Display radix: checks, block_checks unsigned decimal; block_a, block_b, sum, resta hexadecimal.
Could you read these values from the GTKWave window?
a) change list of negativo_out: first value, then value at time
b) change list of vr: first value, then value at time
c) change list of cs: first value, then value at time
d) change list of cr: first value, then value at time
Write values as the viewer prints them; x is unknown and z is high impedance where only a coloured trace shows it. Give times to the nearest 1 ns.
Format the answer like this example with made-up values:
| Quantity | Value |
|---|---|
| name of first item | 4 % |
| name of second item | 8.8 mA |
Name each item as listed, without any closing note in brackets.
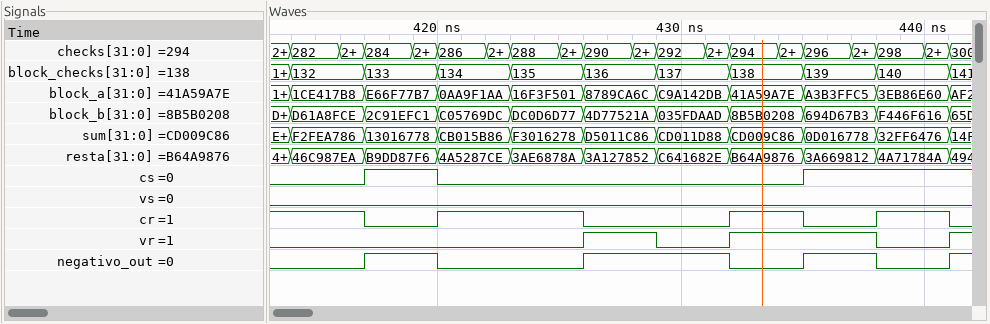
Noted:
| Quantity | Value |
|---|---|
| change list of negativo_out: first value, then value at time | 0, 1 at 417 ns, 0 at 420 ns, 1 at 426 ns, 0 at 432 ns, 1 at 435 ns, 0 at 438 ns, 1 at 441 ns |
| change list of vr: first value, then value at time | 0, 1 at 426 ns, 0 at 429 ns, 1 at 432 ns, 0 at 438 ns, 1 at 441 ns |
| change list of cs: first value, then value at time | 0, 1 at 417 ns, 0 at 420 ns, 1 at 435 ns |
| change list of cr: first value, then value at time | 1, 0 at 417 ns, 1 at 420 ns, 0 at 426 ns, 1 at 432 ns, 0 at 435 ns, 1 at 438 ns, 0 at 441 ns |
